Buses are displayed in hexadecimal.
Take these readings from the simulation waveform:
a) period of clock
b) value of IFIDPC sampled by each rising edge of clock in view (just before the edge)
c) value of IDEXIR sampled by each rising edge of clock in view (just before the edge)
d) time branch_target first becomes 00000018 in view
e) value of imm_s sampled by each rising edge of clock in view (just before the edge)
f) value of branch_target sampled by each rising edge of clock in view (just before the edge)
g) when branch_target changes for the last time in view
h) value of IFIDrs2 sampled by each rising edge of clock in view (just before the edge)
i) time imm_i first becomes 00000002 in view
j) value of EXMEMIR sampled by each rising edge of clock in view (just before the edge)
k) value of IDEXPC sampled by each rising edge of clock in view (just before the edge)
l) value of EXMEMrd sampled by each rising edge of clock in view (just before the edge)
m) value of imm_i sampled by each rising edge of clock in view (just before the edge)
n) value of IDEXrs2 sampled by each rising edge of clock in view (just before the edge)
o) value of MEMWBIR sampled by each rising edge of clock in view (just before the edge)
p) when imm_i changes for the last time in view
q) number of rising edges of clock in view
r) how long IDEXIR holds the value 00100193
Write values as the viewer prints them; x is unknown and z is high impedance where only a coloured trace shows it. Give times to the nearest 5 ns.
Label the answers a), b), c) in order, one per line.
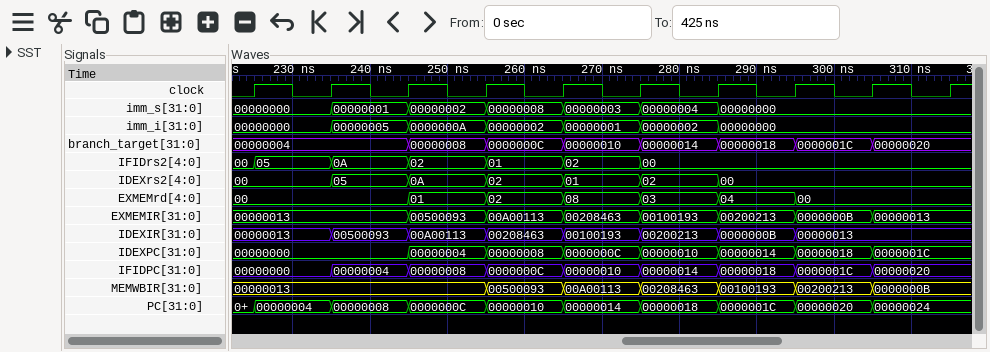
a) 10 ns
b) 00000000, 00000000, 00000004, 00000008, 0000000C, 00000010, 00000014, 00000018, 0000001C, 00000020
c) 00000013, 00000013, 00500093, 00A00113, 00208463, 00100193, 00200213, 0000000B, 00000013, 00000013
d) 285 ns
e) 00000000, 00000000, 00000001, 00000002, 00000008, 00000003, 00000004, 00000000, 00000000, 00000000
f) 00000004, 00000004, 00000004, 00000008, 0000000C, 00000010, 00000014, 00000018, 0000001C, 00000020
g) 305 ns
h) 00, 05, 0A, 02, 01, 02, 00, 00, 00, 00
i) 255 ns
j) 00000013, 00000013, 00000013, 00500093, 00A00113, 00208463, 00100193, 00200213, 0000000B, 00000013
k) 00000000, 00000000, 00000000, 00000004, 00000008, 0000000C, 00000010, 00000014, 00000018, 0000001C
l) 00, 00, 00, 01, 02, 08, 03, 04, 00, 00
m) 00000000, 00000000, 00000005, 0000000A, 00000002, 00000001, 00000002, 00000000, 00000000, 00000000
n) 00, 00, 05, 0A, 02, 01, 02, 00, 00, 00
o) 00000013, 00000013, 00000013, 00000013, 00500093, 00A00113, 00208463, 00100193, 00200213, 0000000B
p) 285 ns
q) 10
r) 10 ns
